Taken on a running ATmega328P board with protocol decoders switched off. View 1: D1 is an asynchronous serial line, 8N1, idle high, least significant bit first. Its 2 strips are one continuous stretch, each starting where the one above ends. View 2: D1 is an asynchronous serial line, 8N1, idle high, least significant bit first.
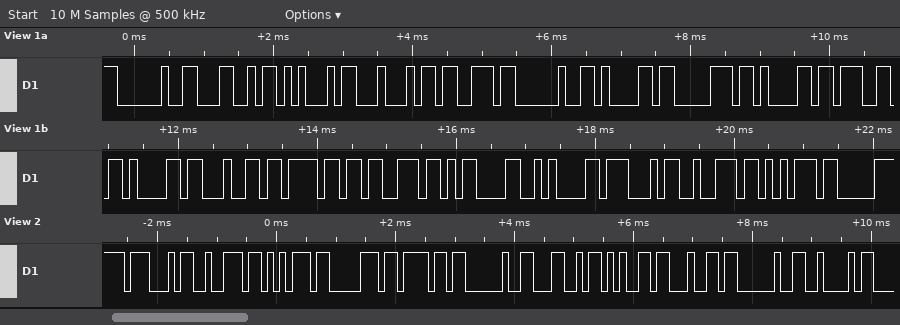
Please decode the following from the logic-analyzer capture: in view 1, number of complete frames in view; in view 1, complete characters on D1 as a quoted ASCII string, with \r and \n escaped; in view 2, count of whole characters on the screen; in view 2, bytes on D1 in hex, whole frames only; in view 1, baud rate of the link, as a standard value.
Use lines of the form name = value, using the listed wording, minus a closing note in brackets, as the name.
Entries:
in view 1, number of complete frames in view = 19
in view 1, complete characters on D1 as a quoted ASCII string, with \r and \n escaped = " LEDs apagados\r\nGru"
in view 2, count of whole characters on the screen = 11
in view 2, bytes on D1 in hex, whole frames only = 47 72 75 70 6F 20 4C 65 64 20 42
in view 1, baud rate of the link, as a standard value = 9600 baud
